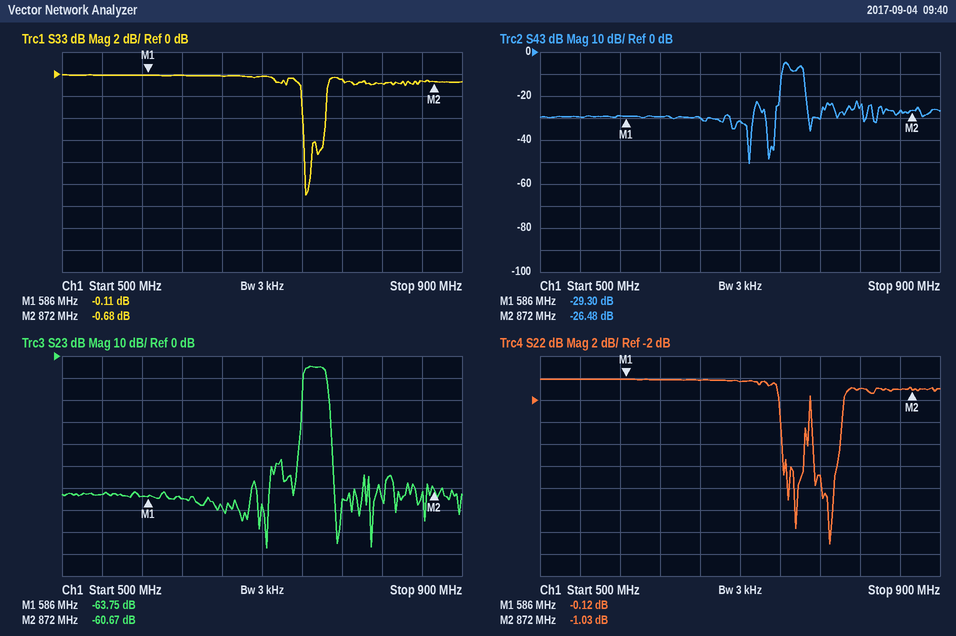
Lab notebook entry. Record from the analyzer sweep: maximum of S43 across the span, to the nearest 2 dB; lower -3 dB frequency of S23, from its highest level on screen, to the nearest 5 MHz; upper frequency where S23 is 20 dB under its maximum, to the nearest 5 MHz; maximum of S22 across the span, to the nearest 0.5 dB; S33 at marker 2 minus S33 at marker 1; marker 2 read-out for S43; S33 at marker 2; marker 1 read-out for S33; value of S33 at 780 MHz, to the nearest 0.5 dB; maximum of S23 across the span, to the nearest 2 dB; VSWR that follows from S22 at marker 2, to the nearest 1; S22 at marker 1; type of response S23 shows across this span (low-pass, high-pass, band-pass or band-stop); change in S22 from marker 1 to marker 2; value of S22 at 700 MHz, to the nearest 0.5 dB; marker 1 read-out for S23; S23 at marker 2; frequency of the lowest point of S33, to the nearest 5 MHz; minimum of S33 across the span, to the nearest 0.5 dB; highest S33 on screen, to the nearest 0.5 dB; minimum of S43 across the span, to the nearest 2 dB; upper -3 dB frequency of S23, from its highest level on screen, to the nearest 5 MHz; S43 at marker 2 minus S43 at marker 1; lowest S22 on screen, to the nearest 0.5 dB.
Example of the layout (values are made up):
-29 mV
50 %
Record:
-4 dB
740 MHz
770 MHz
0.0 dB
-0.57 dB
-26.48 dB
-0.68 dB
-0.11 dB
-0.5 dB
-4 dB
17
-0.12 dB
band-pass
-0.91 dB
-0.5 dB
-63.75 dB
-60.67 dB
745 MHz
-11.0 dB
0.0 dB
-50 dB
765 MHz
2.82 dB
-15.0 dB
